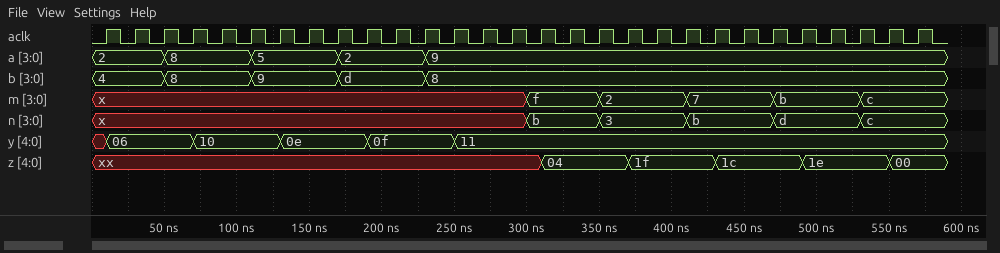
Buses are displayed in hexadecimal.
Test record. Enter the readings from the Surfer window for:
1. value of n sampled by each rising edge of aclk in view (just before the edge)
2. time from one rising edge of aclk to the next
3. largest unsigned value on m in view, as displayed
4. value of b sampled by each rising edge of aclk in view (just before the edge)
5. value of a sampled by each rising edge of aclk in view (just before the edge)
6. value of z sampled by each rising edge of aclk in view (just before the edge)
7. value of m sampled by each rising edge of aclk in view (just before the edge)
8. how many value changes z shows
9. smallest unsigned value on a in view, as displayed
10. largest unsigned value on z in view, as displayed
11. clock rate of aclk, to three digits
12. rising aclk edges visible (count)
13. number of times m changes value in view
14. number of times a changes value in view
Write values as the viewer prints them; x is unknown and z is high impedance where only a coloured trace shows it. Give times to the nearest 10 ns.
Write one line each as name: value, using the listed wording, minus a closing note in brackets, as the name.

value of n sampled by each rising edge of aclk in view: x, x, x, x, x, x, x, x, x, x, x, x, x, x, x, b, b, b, 3, 3, 3, b, b, b, d, d, d, c, c
time from one rising edge of aclk to the next: 20 ns
largest unsigned value on m in view, as displayed: f
value of b sampled by each rising edge of aclk in view: 4, 4, 4, 8, 8, 8, 9, 9, 9, d, d, d, 8, 8, 8, 8, 8, 8, 8, 8, 8, 8, 8, 8, 8, 8, 8, 8, 8
value of a sampled by each rising edge of aclk in view: 2, 2, 2, 8, 8, 8, 5, 5, 5, 2, 2, 2, 9, 9, 9, 9, 9, 9, 9, 9, 9, 9, 9, 9, 9, 9, 9, 9, 9
value of z sampled by each rising edge of aclk in view: xx, xx, xx, xx, xx, xx, xx, xx, xx, xx, xx, xx, xx, xx, xx, xx, 04, 04, 04, 1f, 1f, 1f, 1c, 1c, 1c, 1e, 1e, 1e, 00
value of m sampled by each rising edge of aclk in view: x, x, x, x, x, x, x, x, x, x, x, x, x, x, x, f, f, f, 2, 2, 2, 7, 7, 7, b, b, b, c, c
how many value changes z shows: 5
smallest unsigned value on a in view, as displayed: 2
largest unsigned value on z in view, as displayed: 1f
clock rate of aclk, to three digits: 50.0 MHz
rising aclk edges visible: 29
number of times m changes value in view: 5
number of times a changes value in view: 4
